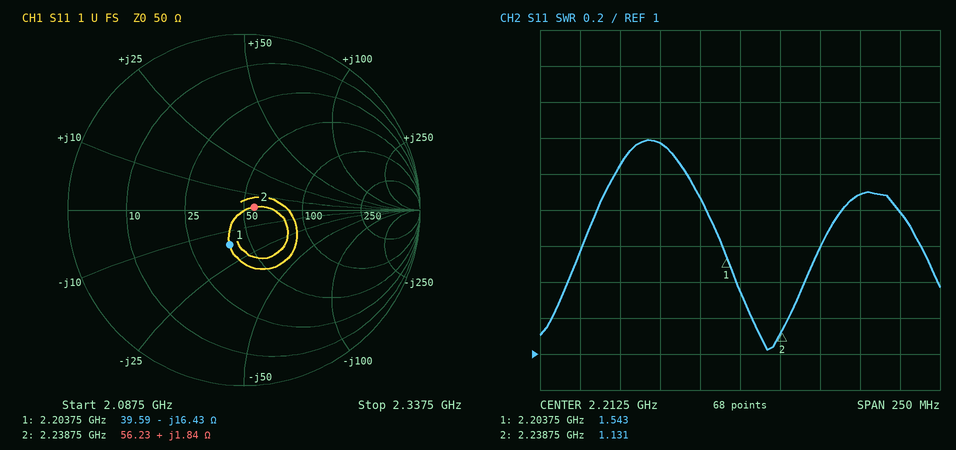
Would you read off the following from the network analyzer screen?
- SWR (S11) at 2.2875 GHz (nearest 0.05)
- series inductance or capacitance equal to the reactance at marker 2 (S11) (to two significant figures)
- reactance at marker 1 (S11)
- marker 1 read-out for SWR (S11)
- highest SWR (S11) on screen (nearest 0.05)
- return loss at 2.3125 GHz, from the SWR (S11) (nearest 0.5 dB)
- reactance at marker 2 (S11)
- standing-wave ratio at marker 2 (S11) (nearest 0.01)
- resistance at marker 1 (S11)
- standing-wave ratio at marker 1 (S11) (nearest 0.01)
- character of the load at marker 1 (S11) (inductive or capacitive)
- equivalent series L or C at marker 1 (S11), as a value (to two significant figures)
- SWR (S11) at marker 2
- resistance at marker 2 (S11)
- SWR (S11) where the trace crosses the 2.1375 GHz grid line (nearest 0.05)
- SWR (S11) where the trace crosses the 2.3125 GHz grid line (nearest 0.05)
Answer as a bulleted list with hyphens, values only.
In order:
- 1.90
- 130 pH
- -16.43 Ω
- 1.543
- 2.20
- 11.0 dB
- +1.84 Ω
- 1.13
- 39.59 Ω
- 1.54
- capacitive
- 4.4 pF
- 1.131
- 56.23 Ω
- 2.05
- 1.80
